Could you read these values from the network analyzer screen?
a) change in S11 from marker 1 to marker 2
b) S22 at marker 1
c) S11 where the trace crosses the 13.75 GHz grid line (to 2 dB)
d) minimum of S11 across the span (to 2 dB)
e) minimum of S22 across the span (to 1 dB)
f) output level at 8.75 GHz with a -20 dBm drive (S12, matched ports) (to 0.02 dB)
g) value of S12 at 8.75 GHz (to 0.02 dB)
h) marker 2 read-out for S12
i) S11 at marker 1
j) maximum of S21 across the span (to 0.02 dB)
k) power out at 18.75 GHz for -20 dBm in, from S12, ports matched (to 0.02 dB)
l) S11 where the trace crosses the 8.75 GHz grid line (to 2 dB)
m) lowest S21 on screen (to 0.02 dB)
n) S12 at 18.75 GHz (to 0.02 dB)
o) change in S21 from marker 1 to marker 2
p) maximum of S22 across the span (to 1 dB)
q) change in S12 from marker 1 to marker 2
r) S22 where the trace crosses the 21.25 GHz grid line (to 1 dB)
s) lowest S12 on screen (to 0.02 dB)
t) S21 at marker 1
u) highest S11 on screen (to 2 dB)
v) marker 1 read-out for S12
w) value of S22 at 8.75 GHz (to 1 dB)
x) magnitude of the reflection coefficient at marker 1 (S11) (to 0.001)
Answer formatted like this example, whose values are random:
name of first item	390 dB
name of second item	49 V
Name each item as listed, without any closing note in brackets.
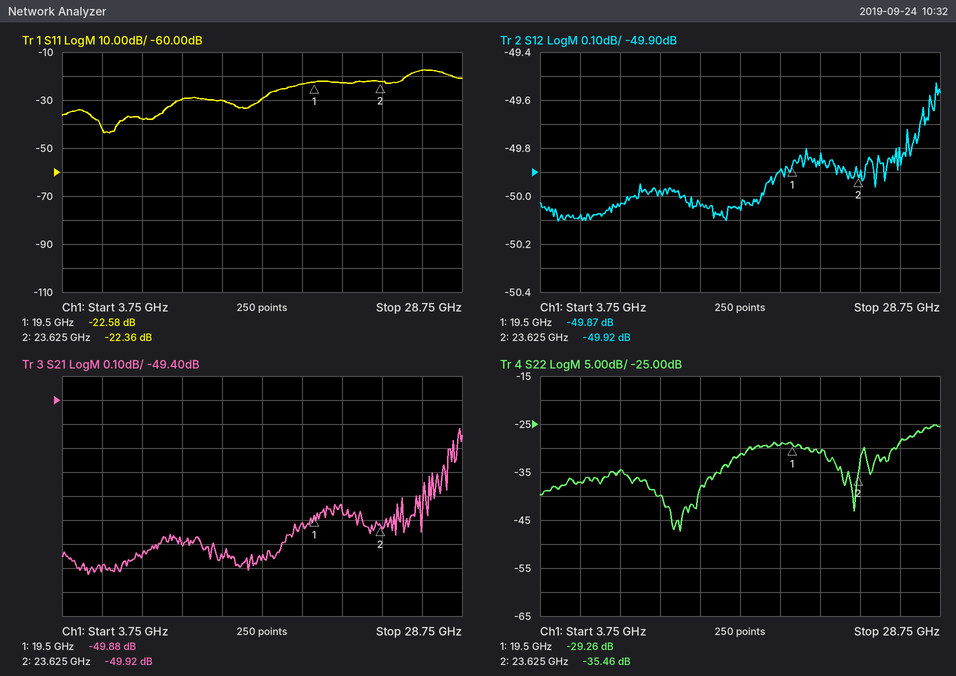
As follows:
change in S11 from marker 1 to marker 2	0.22 dB
S22 at marker 1	-29.26 dB
S11 where the trace crosses the 13.75 GHz grid line	-30 dB
minimum of S11 across the span	-44 dB
minimum of S22 across the span	-47 dB
output level at 8.75 GHz with a -20 dBm drive (S12, matched ports)	-70.04 dBm
value of S12 at 8.75 GHz	-50.04 dB
marker 2 read-out for S12	-49.92 dB
S11 at marker 1	-22.58 dB
maximum of S21 across the span	-49.52 dB
power out at 18.75 GHz for -20 dBm in, from S12, ports matched	-69.90 dBm
S11 where the trace crosses the 8.75 GHz grid line	-38 dB
lowest S21 on screen	-50.12 dB
S12 at 18.75 GHz	-49.90 dB
change in S21 from marker 1 to marker 2	-0.04 dB
maximum of S22 across the span	-25 dB
change in S12 from marker 1 to marker 2	-0.05 dB
S22 where the trace crosses the 21.25 GHz grid line	-31 dB
lowest S12 on screen	-50.10 dB
S21 at marker 1	-49.88 dB
highest S11 on screen	-18 dB
marker 1 read-out for S12	-49.87 dB
value of S22 at 8.75 GHz	-35 dB
magnitude of the reflection coefficient at marker 1 (S11)	0.074
